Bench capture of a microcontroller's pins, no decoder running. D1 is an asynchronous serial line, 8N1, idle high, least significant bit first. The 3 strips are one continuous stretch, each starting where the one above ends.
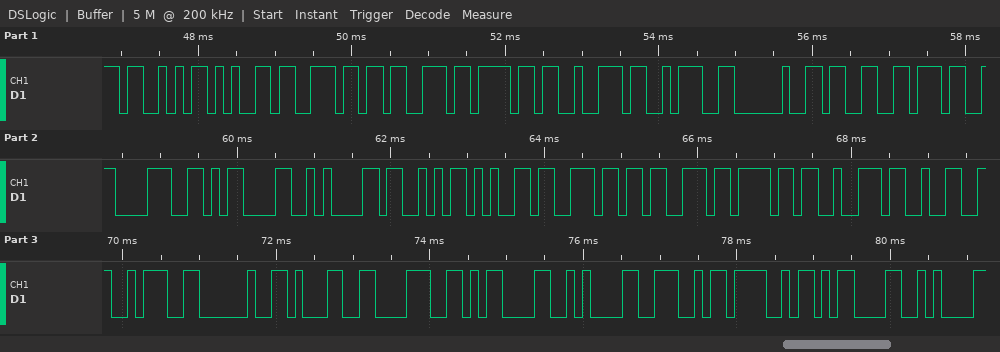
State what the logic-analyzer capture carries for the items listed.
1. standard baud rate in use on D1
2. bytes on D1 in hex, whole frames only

9600 baud
53 65 6E 73 6F 72 3A 20 33 37 38 0D 0A 53 65 6E 73 6F 72 32 3A 20 31 38 0D 0A 4E 4F 0D 0A
